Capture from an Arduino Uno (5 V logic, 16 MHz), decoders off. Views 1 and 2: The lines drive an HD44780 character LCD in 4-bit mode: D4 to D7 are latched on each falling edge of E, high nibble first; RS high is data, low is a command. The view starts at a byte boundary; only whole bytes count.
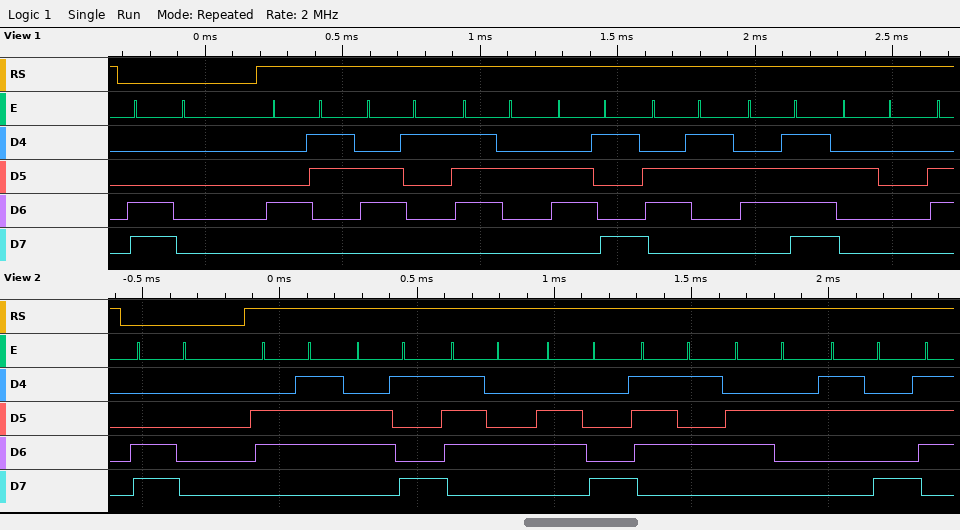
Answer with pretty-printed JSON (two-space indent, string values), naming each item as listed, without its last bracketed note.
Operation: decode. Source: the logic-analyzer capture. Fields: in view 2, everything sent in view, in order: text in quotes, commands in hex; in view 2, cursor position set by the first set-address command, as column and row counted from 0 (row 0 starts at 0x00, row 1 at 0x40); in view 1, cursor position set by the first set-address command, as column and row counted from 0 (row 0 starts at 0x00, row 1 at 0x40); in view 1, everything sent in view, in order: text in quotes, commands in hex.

{
  "in view 2, everything sent in view, in order: text in quotes, commands in hex": "0xC0 \"github:\"",
  "in view 2, cursor position set by the first set-address command, as column and row counted from 0": "column 0, row 1",
  "in view 1, cursor position set by the first set-address command, as column and row counted from 0": "column 0, row 1",
  "in view 1, everything sent in view, in order: text in quotes, commands in hex": "0xC0 \"Carico \""
}
